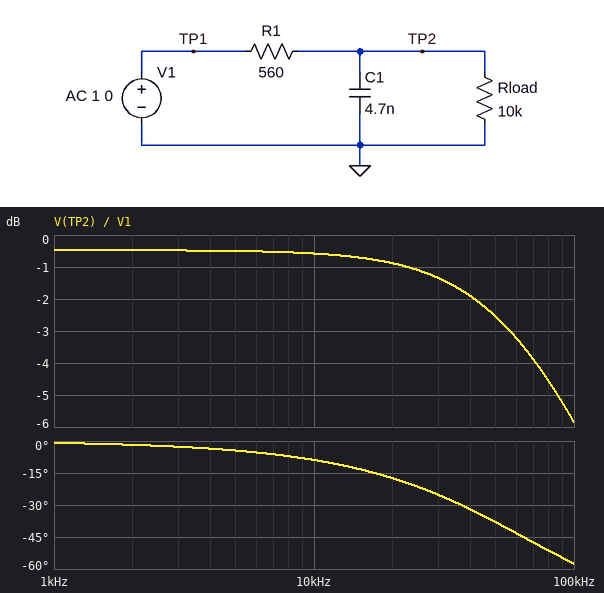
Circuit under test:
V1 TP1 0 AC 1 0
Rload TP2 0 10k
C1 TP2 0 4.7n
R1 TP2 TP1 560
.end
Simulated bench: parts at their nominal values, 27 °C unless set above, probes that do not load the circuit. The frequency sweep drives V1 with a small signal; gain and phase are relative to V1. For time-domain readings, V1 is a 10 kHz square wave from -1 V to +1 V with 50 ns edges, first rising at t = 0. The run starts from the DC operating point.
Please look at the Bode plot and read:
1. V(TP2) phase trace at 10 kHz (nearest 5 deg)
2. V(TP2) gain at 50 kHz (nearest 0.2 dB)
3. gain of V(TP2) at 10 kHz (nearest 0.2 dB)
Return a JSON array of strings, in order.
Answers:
["-10 deg", "-2.6 dB", "-0.6 dB"]
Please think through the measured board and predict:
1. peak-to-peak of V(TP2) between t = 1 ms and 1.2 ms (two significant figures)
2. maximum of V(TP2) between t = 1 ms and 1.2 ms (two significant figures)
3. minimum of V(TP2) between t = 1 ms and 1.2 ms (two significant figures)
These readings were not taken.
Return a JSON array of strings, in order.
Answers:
["1.9 V", "950 mV", "-950 mV"]
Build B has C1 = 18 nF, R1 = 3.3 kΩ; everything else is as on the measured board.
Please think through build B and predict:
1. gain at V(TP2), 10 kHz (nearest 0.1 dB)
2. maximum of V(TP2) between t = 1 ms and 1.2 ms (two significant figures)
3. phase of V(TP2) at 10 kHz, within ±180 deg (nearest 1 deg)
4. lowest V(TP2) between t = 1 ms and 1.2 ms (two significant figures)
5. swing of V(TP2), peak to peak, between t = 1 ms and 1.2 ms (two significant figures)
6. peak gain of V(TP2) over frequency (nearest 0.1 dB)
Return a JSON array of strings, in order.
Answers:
["-12.0 dB", "380 mV", "-70 deg", "-380 mV", "760 mV", "-2.5 dB"]
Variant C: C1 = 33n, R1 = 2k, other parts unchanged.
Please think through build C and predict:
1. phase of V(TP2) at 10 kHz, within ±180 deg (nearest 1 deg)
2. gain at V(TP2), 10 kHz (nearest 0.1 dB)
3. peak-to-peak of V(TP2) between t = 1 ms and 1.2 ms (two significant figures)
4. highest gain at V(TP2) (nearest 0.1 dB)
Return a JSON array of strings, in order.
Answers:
["-74 deg", "-12.7 dB", "710 mV", "-1.6 dB"]
